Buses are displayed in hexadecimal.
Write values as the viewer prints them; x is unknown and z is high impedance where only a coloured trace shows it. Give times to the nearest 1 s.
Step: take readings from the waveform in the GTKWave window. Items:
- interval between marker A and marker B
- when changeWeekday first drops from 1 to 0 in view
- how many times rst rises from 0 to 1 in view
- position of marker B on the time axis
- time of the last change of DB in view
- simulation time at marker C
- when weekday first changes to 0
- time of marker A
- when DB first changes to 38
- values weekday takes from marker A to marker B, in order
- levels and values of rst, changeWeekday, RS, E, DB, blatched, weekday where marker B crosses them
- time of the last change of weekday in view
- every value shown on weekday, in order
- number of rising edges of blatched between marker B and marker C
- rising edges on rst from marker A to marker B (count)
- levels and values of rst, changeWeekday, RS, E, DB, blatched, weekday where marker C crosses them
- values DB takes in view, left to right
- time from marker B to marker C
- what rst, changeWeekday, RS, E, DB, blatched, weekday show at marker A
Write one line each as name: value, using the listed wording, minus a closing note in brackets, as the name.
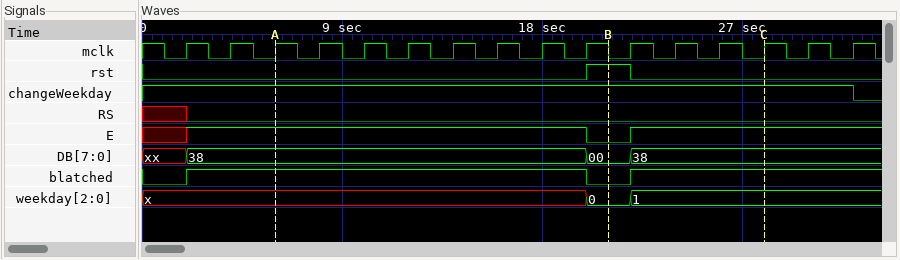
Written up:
interval between marker A and marker B: 15 s
when changeWeekday first drops from 1 to 0 in view: 32 s
how many times rst rises from 0 to 1 in view: 1
position of marker B on the time axis: 21 s
time of the last change of DB in view: 22 s
simulation time at marker C: 28 s
when weekday first changes to 0: 20 s
time of marker A: 6 s
when DB first changes to 38: 2 s
values weekday takes from marker A to marker B, in order: x, 0
levels and values of rst, changeWeekday, RS, E, DB, blatched, weekday where marker B crosses them: rst=1, changeWeekday=1, RS=0, E=0, DB=00, blatched=0, weekday=0
time of the last change of weekday in view: 22 s
every value shown on weekday, in order: x, 0, 1
number of rising edges of blatched between marker B and marker C: 1
rising edges on rst from marker A to marker B: 1
levels and values of rst, changeWeekday, RS, E, DB, blatched, weekday where marker C crosses them: rst=0, changeWeekday=1, RS=0, E=1, DB=38, blatched=1, weekday=1
values DB takes in view, left to right: xx, 38, 00, 38
time from marker B to marker C: 7 s
what rst, changeWeekday, RS, E, DB, blatched, weekday show at marker A: rst=0, changeWeekday=1, RS=0, E=1, DB=38, blatched=1, weekday=x
